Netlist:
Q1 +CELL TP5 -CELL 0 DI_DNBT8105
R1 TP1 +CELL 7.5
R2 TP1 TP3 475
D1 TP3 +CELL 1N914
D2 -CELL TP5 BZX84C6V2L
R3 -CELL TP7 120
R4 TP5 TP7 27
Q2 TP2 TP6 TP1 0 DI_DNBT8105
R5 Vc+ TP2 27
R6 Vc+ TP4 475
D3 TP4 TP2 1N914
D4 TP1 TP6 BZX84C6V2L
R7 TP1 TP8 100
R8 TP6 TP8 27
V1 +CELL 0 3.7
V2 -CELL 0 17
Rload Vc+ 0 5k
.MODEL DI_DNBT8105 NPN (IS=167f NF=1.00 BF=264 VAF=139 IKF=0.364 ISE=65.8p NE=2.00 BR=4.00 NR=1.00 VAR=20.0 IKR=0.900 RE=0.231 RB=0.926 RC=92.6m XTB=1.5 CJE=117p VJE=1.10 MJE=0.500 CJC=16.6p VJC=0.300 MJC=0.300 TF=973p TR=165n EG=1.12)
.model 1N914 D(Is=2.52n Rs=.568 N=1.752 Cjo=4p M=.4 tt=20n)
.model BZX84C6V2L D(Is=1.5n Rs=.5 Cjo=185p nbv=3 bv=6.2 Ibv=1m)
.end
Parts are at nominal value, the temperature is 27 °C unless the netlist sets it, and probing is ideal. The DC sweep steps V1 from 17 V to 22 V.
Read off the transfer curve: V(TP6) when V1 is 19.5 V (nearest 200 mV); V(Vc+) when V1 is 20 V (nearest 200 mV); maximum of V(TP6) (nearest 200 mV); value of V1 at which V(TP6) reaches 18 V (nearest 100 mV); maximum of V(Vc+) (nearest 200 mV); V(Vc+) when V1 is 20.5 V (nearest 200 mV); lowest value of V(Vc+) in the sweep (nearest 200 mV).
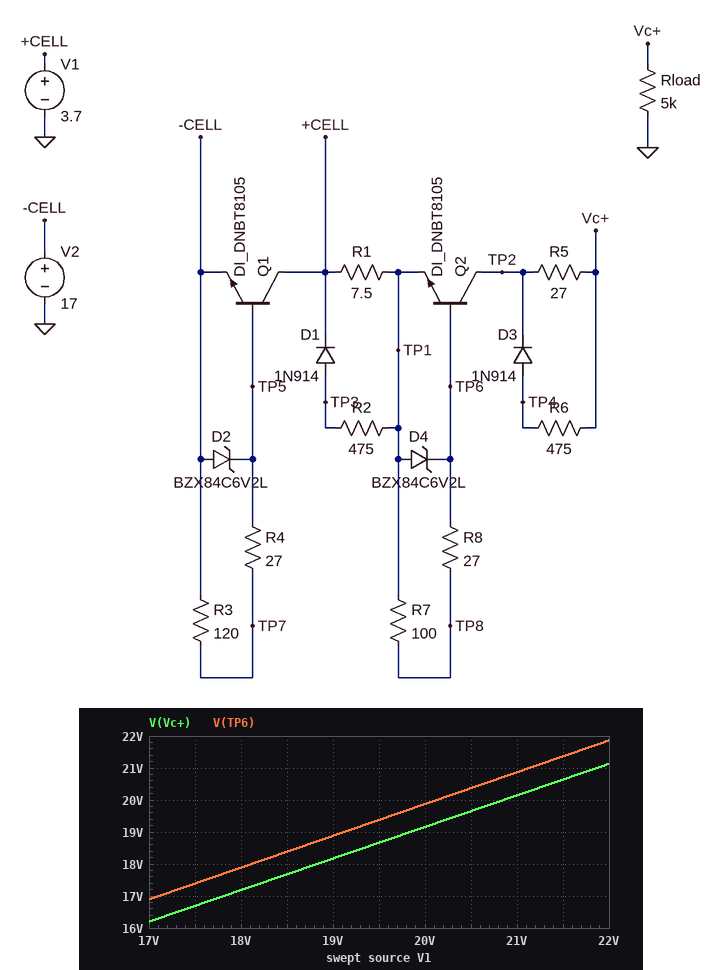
19.4 V
19.2 V
21.8 V
18.1 V
21.2 V
19.6 V
16.2 V
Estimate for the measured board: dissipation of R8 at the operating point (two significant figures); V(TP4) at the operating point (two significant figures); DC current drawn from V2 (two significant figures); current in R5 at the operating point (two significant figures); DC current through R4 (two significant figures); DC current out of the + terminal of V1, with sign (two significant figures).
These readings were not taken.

420 nW
3.1 V
14 A
620 µA
29 mA
-14 A
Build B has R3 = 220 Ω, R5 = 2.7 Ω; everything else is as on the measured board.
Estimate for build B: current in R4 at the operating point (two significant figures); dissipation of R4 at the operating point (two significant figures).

17 mA
8.1 mW
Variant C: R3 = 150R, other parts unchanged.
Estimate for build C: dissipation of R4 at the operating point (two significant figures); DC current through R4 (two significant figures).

16 mW
24 mA
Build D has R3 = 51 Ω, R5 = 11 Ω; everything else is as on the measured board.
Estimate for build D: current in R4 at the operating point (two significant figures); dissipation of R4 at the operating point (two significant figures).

55 mA
80 mW
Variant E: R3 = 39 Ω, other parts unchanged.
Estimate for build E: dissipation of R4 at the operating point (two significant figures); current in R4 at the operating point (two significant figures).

110 mW
64 mA
